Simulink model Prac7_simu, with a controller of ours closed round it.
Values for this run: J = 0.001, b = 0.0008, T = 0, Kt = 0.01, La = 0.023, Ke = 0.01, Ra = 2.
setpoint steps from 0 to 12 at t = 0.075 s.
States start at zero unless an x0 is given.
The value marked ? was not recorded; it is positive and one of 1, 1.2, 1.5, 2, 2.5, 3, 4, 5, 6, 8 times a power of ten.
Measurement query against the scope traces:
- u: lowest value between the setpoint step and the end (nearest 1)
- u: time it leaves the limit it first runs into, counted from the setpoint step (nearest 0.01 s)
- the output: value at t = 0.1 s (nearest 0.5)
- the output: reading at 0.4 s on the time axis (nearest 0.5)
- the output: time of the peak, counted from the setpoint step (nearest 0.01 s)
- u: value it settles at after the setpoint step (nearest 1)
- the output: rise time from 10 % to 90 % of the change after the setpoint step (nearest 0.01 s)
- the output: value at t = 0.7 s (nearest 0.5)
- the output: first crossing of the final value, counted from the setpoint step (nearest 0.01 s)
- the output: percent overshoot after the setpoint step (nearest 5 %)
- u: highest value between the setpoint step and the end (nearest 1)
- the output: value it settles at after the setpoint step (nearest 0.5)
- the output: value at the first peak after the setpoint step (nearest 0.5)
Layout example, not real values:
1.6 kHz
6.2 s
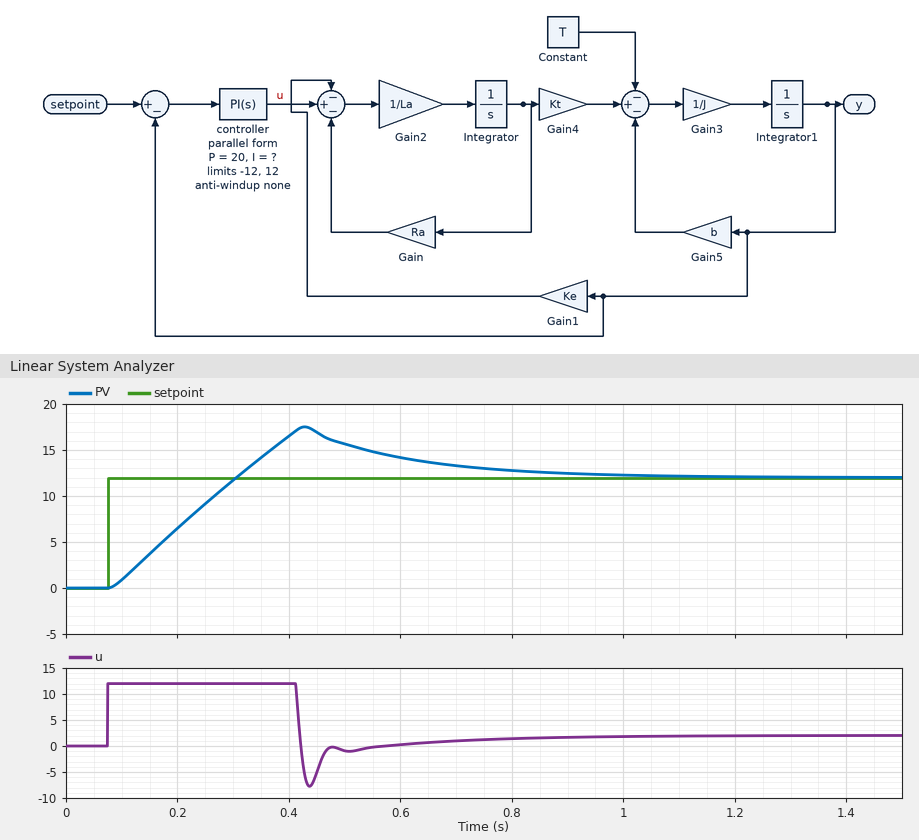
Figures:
-8
0.34 s
1.0
16.5
0.35 s
2
0.18 s
13.5
0.23 s
45 %
12
12.0
17.5
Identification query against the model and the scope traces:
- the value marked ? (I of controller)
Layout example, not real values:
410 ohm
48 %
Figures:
100
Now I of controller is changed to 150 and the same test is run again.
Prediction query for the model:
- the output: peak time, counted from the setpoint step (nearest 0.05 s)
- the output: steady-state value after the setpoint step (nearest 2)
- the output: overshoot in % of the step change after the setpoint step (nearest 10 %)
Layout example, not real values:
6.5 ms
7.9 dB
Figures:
0.40 s
12
60 %
